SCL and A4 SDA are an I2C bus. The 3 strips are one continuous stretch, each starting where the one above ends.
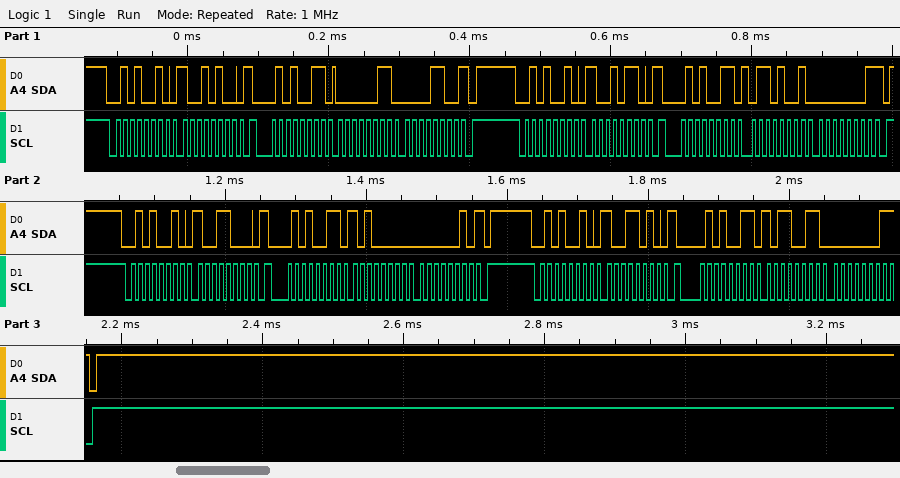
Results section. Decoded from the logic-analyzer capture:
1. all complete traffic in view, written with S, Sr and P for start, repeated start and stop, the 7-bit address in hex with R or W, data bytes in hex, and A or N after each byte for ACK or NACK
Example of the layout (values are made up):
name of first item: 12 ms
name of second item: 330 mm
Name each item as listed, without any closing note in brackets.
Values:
all complete traffic in view, written with S, Sr and P for start, repeated start and stop, the 7-bit address in hex with R or W, data bytes in hex, and A or N after each byte for ACK or NACK: S 29W A 94 A Sr 29R A 03 A 0C N P S 29W A 96 A Sr 29R A 69 A 01 N P S 29W A 98 A Sr 29R A A0 A 02 N P S 29W A 9A A Sr 29R A B3 A 01 N P
